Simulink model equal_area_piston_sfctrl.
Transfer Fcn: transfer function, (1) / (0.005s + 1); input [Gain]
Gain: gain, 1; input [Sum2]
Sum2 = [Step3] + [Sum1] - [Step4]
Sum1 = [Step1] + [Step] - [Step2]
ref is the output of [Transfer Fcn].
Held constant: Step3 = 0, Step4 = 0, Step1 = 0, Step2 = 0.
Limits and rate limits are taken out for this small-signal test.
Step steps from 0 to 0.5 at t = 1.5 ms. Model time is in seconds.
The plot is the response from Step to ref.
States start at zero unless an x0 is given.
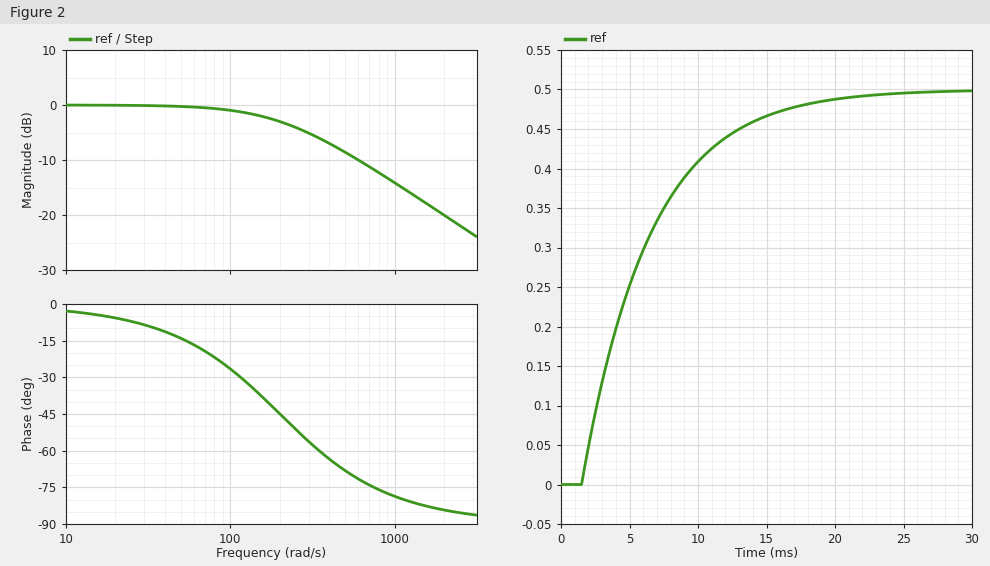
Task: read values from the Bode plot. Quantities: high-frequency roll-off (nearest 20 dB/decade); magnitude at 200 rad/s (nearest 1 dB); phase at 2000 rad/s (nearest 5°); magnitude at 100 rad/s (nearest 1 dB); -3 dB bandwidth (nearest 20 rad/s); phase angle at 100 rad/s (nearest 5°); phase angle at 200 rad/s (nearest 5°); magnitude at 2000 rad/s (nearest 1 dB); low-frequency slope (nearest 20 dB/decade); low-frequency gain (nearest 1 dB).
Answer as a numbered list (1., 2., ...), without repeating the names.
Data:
1. -20 dB/decade
2. -3 dB
3. -85°
4. -1 dB
5. 200 rad/s
6. -25°
7. -45°
8. -20 dB
9. 0 dB/decade
10. 0 dB
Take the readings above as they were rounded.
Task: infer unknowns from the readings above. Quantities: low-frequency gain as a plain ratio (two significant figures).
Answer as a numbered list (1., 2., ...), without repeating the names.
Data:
1. 1.0
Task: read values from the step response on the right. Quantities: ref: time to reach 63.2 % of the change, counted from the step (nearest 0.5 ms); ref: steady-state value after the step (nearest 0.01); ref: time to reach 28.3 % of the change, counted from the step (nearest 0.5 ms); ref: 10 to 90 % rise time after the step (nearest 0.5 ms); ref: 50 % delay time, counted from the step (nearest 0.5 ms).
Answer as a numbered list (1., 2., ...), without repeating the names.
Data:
1. 5.0 ms
2. 0.50
3. 1.5 ms
4. 11.0 ms
5. 3.5 ms
